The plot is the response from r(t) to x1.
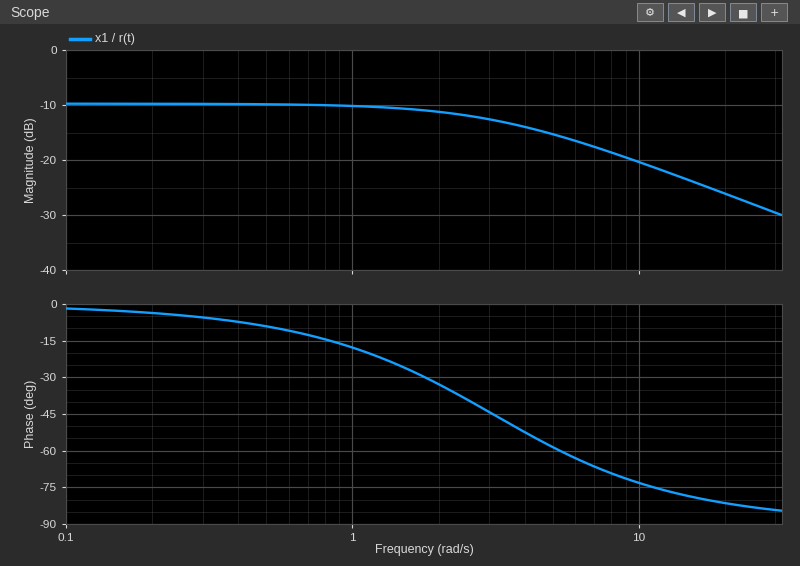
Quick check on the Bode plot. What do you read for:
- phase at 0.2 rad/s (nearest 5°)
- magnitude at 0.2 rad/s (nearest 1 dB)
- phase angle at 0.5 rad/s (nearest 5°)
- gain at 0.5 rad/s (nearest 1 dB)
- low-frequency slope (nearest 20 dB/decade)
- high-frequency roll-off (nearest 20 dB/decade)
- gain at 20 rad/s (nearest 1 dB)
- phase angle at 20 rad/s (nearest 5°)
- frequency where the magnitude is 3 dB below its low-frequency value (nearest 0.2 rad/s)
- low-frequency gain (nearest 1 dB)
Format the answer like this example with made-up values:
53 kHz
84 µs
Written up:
-5°
-10 dB
-10°
-10 dB
0 dB/decade
-20 dB/decade
-26 dB
-80°
3.2 rad/s
-10 dB
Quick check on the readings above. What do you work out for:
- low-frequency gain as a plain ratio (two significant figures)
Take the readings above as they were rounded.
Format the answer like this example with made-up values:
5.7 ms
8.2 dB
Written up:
0.32
